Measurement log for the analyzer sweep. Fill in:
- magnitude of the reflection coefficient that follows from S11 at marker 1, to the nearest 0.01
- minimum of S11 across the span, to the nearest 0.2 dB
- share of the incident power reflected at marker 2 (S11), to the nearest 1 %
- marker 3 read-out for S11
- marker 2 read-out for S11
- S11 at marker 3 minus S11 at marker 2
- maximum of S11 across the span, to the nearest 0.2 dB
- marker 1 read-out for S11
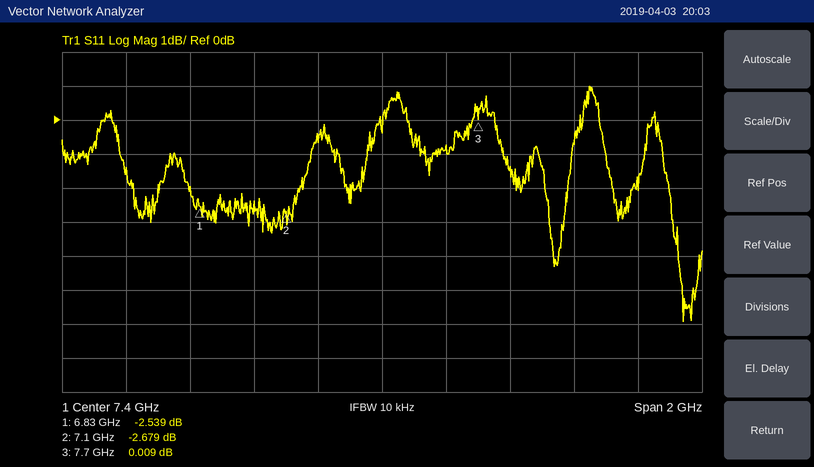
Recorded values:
0.75
-6.0 dB
54 %
0.009 dB
-2.679 dB
2.688 dB
1.0 dB
-2.539 dB
